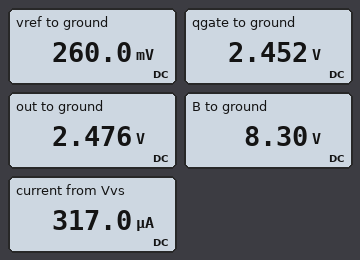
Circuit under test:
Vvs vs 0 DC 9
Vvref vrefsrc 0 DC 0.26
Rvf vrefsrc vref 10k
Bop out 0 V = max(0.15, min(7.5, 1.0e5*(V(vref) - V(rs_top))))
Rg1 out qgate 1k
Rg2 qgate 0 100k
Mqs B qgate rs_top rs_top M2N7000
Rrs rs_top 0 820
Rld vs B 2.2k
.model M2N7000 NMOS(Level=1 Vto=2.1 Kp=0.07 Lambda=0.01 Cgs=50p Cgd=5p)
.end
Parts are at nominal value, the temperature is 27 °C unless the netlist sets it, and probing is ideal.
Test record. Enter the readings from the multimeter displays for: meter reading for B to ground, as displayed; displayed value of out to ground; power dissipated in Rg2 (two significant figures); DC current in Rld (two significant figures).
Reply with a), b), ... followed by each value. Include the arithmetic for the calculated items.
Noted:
a) 8.30 V
b) 2.476 V
c) (2.452 V)^2 / 100 kΩ = 60 µW
d) (9 V - 8.3 V) / 2.2 kΩ = 320 µA
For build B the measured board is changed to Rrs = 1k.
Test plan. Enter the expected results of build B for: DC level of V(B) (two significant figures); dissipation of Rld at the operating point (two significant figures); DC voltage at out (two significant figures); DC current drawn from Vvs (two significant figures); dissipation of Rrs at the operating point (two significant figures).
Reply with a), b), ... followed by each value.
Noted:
a) 8.4 V
b) 150 µW
c) 2.5 V
d) 260 µA
e) 68 µW
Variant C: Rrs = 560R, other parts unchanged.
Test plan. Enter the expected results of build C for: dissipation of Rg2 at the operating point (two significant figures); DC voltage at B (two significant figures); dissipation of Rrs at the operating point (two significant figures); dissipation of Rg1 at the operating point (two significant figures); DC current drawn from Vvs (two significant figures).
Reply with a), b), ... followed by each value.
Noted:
a) 61 µW
b) 8.0 V
c) 120 µW
d) 610 nW
e) 460 µA
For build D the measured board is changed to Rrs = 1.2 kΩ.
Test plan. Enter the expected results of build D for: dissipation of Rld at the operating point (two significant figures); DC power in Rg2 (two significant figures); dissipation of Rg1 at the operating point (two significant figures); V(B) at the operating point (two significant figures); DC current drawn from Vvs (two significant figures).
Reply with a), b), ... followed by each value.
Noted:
a) 100 µW
b) 59 µW
c) 590 nW
d) 8.5 V
e) 220 µA
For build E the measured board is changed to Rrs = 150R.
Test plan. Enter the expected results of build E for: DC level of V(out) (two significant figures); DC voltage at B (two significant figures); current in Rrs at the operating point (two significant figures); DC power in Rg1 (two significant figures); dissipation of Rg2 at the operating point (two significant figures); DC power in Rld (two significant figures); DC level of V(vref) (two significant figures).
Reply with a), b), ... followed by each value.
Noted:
a) 2.6 V
b) 5.2 V
c) 1.7 mA
d) 660 nW
e) 66 µW
f) 6.6 mW
g) 260 mV
